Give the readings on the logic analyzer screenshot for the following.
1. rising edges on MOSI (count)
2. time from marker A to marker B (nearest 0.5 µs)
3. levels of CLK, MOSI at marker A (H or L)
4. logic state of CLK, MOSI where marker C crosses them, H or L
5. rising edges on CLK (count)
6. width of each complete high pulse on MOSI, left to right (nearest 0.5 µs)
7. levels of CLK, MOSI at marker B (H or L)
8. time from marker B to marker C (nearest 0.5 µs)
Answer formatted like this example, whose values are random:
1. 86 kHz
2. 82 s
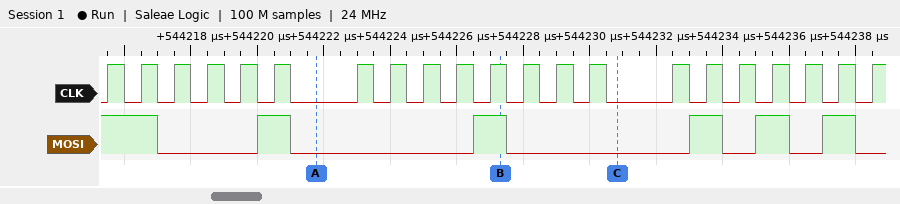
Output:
1. 5
2. 5.5 µs
3. CLK=L, MOSI=L
4. CLK=L, MOSI=L
5. 21
6. 1 µs, 1 µs, 1 µs, 1 µs, 1 µs
7. CLK=H, MOSI=H
8. 3.5 µs
